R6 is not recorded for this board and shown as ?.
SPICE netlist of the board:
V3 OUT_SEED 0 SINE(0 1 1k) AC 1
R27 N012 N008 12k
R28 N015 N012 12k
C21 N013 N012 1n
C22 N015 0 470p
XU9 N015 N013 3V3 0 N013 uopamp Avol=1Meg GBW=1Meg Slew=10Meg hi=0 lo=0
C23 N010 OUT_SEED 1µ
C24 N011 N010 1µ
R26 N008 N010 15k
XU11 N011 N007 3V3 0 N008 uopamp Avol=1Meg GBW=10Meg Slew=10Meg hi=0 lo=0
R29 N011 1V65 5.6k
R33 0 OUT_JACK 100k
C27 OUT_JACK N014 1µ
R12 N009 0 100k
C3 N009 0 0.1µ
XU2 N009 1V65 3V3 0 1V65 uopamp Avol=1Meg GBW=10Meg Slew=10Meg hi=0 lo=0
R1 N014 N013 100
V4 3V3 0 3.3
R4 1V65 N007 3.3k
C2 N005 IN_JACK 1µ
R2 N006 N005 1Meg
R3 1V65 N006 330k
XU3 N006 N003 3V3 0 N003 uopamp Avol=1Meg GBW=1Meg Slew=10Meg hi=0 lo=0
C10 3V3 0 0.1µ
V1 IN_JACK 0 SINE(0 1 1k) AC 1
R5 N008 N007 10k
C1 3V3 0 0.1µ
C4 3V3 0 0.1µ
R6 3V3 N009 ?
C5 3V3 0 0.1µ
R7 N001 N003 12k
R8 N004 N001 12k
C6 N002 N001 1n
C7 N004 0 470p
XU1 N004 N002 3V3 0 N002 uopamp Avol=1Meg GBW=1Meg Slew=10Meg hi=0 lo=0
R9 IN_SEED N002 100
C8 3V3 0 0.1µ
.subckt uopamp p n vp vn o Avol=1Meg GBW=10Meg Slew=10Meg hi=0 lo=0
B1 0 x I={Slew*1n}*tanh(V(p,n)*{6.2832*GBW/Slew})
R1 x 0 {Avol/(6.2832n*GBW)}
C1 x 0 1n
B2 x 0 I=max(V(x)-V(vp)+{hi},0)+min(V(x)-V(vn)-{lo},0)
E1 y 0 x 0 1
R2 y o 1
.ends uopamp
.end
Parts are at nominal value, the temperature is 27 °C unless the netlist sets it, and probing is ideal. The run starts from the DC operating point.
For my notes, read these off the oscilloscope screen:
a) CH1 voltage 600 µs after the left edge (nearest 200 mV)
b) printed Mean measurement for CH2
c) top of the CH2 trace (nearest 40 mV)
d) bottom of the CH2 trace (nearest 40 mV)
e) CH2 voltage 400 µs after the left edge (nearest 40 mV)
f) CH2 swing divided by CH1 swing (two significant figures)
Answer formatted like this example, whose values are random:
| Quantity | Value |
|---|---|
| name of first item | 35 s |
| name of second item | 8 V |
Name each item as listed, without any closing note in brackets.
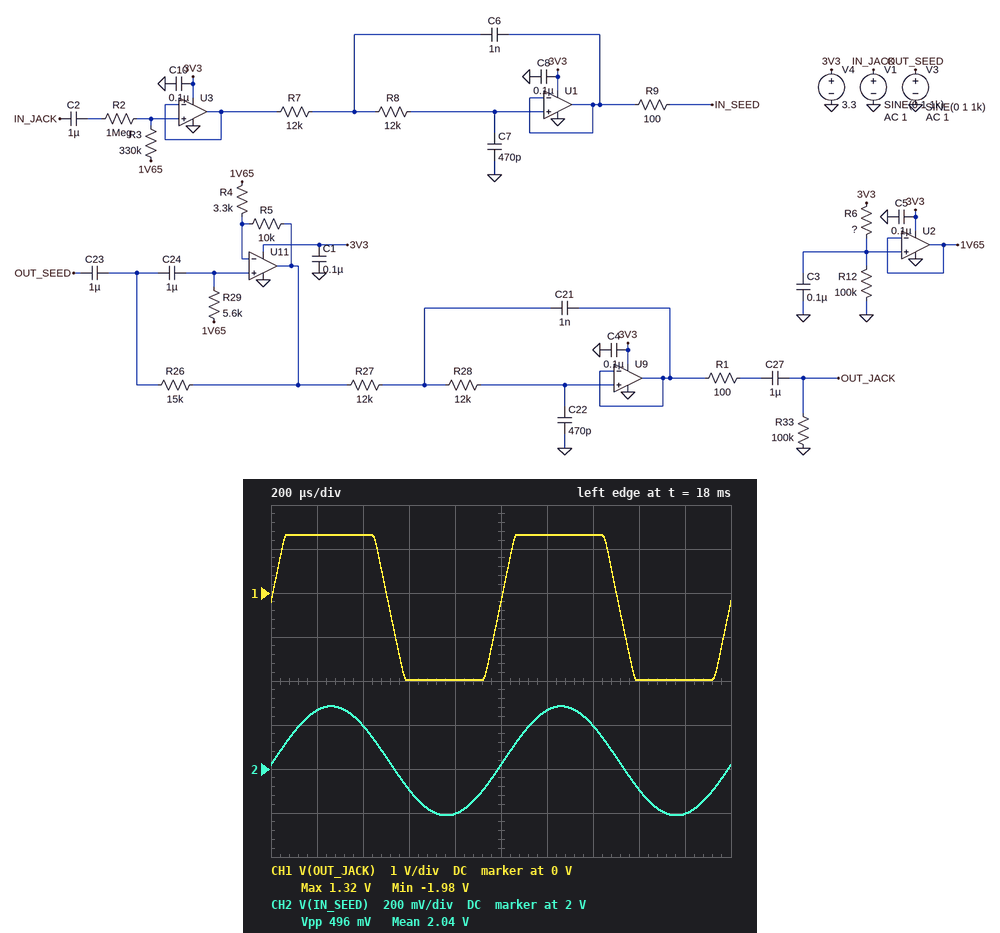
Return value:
| Quantity | Value |
|---|---|
| CH1 voltage 600 µs after the left edge | -2.0 V |
| printed Mean measurement for CH2 | 2.04 V |
| top of the CH2 trace | 2.28 V |
| bottom of the CH2 trace | 1.80 V |
| CH2 voltage 400 µs after the left edge | 2.20 V |
| CH2 swing divided by CH1 swing | 0.15 |
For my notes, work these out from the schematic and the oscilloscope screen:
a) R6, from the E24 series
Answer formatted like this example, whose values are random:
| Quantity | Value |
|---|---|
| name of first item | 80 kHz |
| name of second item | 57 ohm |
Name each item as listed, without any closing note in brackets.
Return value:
| Quantity | Value |
|---|---|
| R6, from the E24 series | 62 kΩ |
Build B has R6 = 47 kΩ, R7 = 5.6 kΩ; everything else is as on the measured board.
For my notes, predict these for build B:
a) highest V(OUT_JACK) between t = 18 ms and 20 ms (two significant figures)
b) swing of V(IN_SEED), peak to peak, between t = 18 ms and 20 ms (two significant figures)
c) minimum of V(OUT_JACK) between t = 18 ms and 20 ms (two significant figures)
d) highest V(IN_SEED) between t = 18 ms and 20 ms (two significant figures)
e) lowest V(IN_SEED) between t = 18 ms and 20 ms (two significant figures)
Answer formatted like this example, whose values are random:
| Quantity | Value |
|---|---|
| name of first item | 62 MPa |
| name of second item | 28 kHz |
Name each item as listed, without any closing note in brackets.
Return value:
| Quantity | Value |
|---|---|
| highest V(OUT_JACK) between t = 18 ms and 20 ms | 1.1 V |
| swing of V(IN_SEED), peak to peak, between t = 18 ms and 20 ms | 500 mV |
| minimum of V(OUT_JACK) between t = 18 ms and 20 ms | -2.2 V |
| highest V(IN_SEED) between t = 18 ms and 20 ms | 2.5 V |
| lowest V(IN_SEED) between t = 18 ms and 20 ms | 2.0 V |
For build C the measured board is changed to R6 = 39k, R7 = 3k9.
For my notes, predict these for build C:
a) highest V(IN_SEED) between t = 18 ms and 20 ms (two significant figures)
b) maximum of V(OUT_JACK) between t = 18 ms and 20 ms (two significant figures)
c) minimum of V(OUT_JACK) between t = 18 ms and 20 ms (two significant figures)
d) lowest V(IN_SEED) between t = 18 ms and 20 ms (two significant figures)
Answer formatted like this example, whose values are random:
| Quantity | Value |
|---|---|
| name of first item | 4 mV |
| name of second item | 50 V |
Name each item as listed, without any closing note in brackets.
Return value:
| Quantity | Value |
|---|---|
| highest V(IN_SEED) between t = 18 ms and 20 ms | 2.6 V |
| maximum of V(OUT_JACK) between t = 18 ms and 20 ms | 1.0 V |
| minimum of V(OUT_JACK) between t = 18 ms and 20 ms | -2.3 V |
| lowest V(IN_SEED) between t = 18 ms and 20 ms | 2.1 V |
